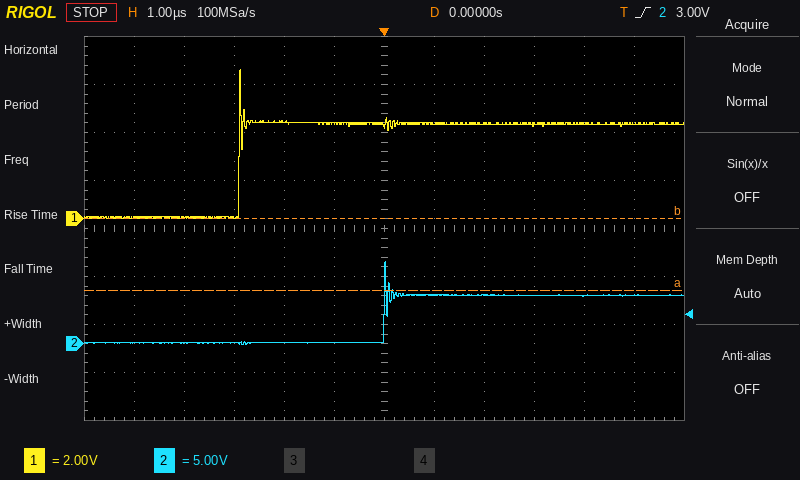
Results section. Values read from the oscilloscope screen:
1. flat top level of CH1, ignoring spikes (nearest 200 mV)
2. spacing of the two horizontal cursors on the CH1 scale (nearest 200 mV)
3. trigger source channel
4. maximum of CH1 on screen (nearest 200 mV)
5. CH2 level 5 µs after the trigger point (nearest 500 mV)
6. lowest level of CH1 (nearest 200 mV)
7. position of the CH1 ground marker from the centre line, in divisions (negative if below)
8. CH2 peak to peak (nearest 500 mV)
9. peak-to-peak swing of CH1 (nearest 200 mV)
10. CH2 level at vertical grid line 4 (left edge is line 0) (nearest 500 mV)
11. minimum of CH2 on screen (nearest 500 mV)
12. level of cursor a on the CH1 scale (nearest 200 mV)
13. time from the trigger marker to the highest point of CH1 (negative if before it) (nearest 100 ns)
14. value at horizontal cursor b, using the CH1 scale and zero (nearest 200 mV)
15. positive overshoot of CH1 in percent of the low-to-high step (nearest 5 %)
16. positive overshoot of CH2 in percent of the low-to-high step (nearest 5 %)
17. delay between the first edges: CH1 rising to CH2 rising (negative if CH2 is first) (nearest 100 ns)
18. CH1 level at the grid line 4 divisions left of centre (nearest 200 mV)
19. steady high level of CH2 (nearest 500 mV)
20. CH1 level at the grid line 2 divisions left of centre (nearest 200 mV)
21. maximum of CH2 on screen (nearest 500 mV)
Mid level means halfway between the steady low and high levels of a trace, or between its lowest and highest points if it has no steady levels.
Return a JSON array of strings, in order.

["4.0 V", "3.0 V", "CH2", "6.2 V", "5.0 V", "0.0 V", "+0.2 div", "8.5 V", "6.2 V", "0.0 V", "0.0 V", "-3.0 V", "-2.9 µs", "0.0 V", "60 %", "70 %", "+2.9 µs", "0.0 V", "5.0 V", "4.0 V", "8.5 V"]
